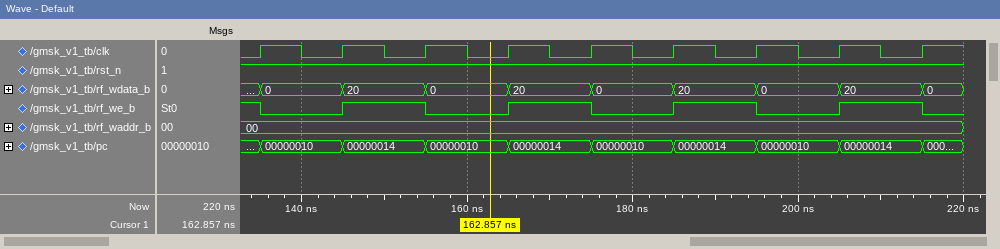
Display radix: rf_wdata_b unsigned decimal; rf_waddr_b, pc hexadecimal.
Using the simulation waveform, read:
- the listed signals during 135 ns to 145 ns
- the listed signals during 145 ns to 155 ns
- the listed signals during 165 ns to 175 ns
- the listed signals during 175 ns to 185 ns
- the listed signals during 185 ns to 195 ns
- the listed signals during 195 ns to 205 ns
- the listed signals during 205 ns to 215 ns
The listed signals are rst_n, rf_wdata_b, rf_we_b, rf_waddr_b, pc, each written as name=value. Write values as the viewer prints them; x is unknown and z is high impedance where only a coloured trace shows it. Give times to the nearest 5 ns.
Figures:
rst_n=1, rf_wdata_b=0, rf_we_b=0, rf_waddr_b=00, pc=00000010
rst_n=1, rf_wdata_b=20, rf_we_b=1, rf_waddr_b=00, pc=00000014
rst_n=1, rf_wdata_b=20, rf_we_b=1, rf_waddr_b=00, pc=00000014
rst_n=1, rf_wdata_b=0, rf_we_b=0, rf_waddr_b=00, pc=00000010
rst_n=1, rf_wdata_b=20, rf_we_b=1, rf_waddr_b=00, pc=00000014
rst_n=1, rf_wdata_b=0, rf_we_b=0, rf_waddr_b=00, pc=00000010
rst_n=1, rf_wdata_b=20, rf_we_b=1, rf_waddr_b=00, pc=00000014
